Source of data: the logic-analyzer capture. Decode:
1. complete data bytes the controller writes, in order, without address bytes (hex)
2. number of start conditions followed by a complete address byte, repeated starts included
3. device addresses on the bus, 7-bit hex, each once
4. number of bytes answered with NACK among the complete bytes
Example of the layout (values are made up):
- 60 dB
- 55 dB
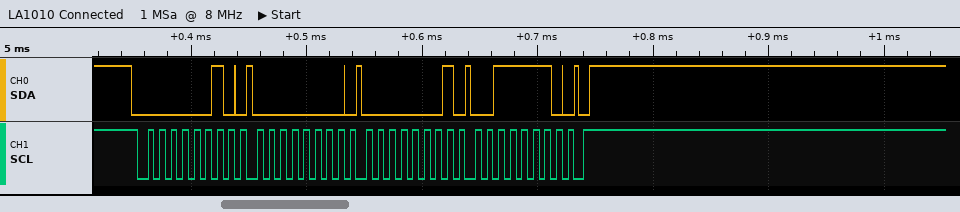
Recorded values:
- 00 01 3E
- 1
- 0x01
- 0
